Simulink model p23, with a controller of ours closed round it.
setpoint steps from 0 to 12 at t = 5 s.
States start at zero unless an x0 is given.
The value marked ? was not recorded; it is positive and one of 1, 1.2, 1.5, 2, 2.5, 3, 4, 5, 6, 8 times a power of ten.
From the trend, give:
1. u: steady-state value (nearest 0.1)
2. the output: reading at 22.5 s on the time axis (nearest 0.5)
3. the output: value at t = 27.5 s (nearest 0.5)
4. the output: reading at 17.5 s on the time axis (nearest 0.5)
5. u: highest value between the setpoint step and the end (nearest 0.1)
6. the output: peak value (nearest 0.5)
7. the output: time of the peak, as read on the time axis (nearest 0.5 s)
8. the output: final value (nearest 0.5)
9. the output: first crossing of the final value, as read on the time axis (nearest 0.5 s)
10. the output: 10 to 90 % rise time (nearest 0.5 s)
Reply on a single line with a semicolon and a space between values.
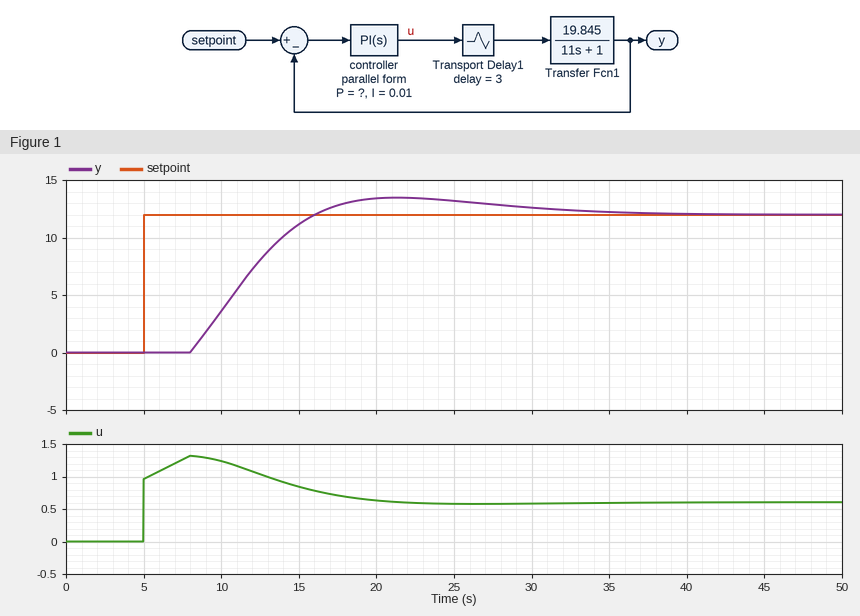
0.6; 13.5; 13.0; 13.0; 1.3; 13.5; 21.5 s; 12.0; 16.0 s; 6.0 s
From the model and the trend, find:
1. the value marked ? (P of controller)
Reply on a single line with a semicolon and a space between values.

0.08
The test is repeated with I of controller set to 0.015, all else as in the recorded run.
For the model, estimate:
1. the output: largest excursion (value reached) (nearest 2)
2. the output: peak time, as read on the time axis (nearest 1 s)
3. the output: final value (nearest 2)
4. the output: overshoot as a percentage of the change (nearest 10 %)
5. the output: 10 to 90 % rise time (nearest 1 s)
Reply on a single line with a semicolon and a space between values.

16; 20 s; 12; 30 %; 5 s
